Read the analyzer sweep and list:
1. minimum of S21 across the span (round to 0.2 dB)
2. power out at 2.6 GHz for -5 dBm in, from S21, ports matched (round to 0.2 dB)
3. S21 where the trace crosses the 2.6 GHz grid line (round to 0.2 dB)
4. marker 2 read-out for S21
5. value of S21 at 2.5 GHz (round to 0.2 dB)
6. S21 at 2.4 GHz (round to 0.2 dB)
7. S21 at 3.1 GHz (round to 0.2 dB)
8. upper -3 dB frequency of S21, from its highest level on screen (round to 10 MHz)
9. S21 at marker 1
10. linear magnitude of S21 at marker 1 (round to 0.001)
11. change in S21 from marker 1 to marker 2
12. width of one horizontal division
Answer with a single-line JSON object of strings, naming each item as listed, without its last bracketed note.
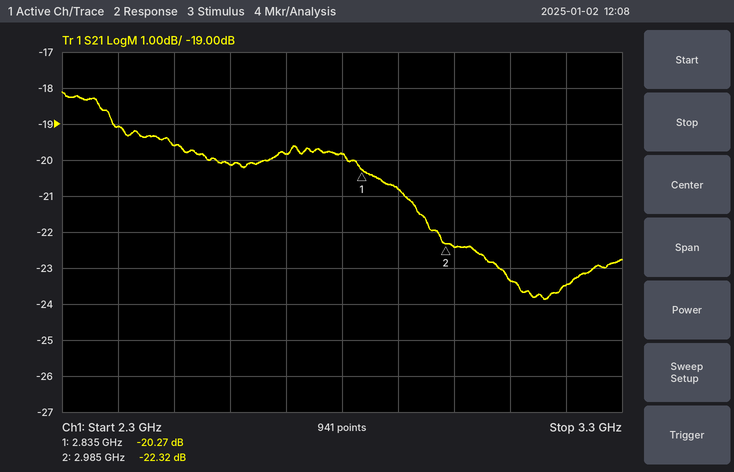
{"minimum of S21 across the span": "-23.8 dB", "power out at 2.6 GHz for -5 dBm in, from S21, ports matched": "-25.2 dBm", "S21 where the trace crosses the 2.6 GHz grid line": "-20.2 dB", "marker 2 read-out for S21": "-22.32 dB", "value of S21 at 2.5 GHz": "-19.6 dB", "S21 at 2.4 GHz": "-19.0 dB", "S21 at 3.1 GHz": "-23.4 dB", "upper -3 dB frequency of S21, from its highest level on screen": "2.92 GHz", "S21 at marker 1": "-20.27 dB", "linear magnitude of S21 at marker 1": "0.097", "change in S21 from marker 1 to marker 2": "-2.05 dB", "width of one horizontal division": "100 MHz"}
